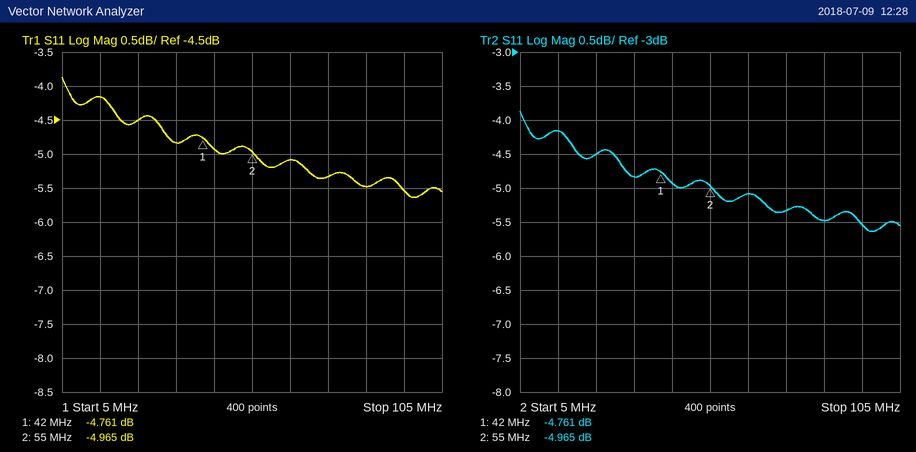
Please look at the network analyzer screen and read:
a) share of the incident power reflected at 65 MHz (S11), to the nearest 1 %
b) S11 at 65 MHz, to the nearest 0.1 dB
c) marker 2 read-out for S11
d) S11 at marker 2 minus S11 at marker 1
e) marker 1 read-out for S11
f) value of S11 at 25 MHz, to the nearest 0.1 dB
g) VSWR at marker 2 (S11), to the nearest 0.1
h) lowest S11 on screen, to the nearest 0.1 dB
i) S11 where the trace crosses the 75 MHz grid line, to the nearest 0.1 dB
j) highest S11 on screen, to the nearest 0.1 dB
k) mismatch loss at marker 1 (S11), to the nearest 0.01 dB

31 %
-5.1 dB
-4.965 dB
-0.204 dB
-4.761 dB
-4.5 dB
3.6
-5.6 dB
-5.3 dB
-3.9 dB
1.77 dB
